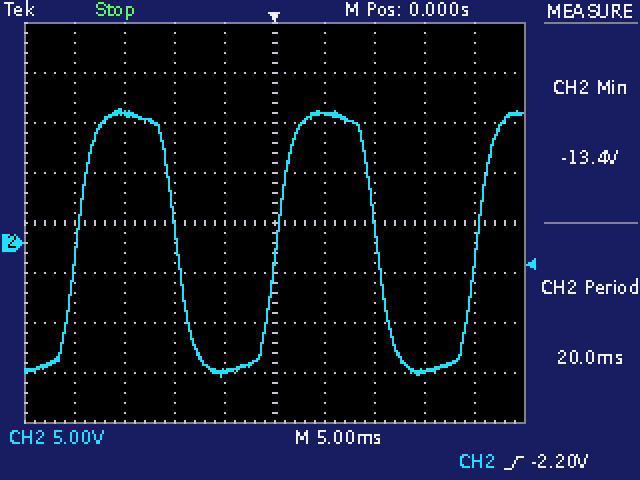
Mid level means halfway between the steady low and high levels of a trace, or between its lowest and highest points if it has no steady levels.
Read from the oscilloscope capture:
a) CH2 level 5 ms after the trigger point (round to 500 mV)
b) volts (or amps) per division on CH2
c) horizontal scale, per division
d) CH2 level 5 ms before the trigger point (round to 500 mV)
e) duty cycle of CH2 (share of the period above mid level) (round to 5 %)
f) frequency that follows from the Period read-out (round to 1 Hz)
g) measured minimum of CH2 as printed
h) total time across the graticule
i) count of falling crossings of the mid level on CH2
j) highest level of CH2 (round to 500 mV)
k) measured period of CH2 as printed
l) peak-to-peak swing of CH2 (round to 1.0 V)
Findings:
13.0 V
5 V
5 ms
-13.0 V
50 %
50 Hz
-13.4 V
50 ms
2
13.5 V
20.0 ms
27.0 V
